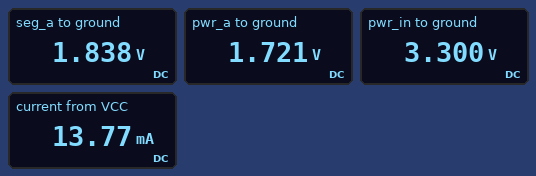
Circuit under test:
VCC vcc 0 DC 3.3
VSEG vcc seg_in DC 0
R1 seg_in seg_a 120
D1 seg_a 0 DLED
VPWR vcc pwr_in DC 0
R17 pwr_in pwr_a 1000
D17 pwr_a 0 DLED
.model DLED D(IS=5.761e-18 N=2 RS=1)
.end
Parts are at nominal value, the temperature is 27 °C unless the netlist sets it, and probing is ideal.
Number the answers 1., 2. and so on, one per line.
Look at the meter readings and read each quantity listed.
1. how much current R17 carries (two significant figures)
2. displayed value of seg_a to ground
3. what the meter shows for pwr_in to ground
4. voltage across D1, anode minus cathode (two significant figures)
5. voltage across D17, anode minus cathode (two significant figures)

1. 1.6 mA
2. 1.838 V
3. 3.300 V
4. 1.8 V
5. 1.7 V
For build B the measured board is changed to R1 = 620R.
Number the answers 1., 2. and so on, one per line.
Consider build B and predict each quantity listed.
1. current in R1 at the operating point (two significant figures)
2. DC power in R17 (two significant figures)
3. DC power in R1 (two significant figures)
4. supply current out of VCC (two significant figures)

1. 2.5 mA
2. 2.5 mW
3. 3.9 mW
4. 4.1 mA
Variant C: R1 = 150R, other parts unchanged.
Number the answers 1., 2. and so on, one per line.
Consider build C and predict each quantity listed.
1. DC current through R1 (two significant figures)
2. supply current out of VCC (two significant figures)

1. 9.8 mA
2. 11 mA
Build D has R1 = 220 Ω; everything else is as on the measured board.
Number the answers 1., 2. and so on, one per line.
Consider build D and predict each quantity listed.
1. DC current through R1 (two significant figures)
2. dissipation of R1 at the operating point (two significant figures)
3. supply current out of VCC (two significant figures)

1. 6.8 mA
2. 10 mW
3. 8.4 mA
